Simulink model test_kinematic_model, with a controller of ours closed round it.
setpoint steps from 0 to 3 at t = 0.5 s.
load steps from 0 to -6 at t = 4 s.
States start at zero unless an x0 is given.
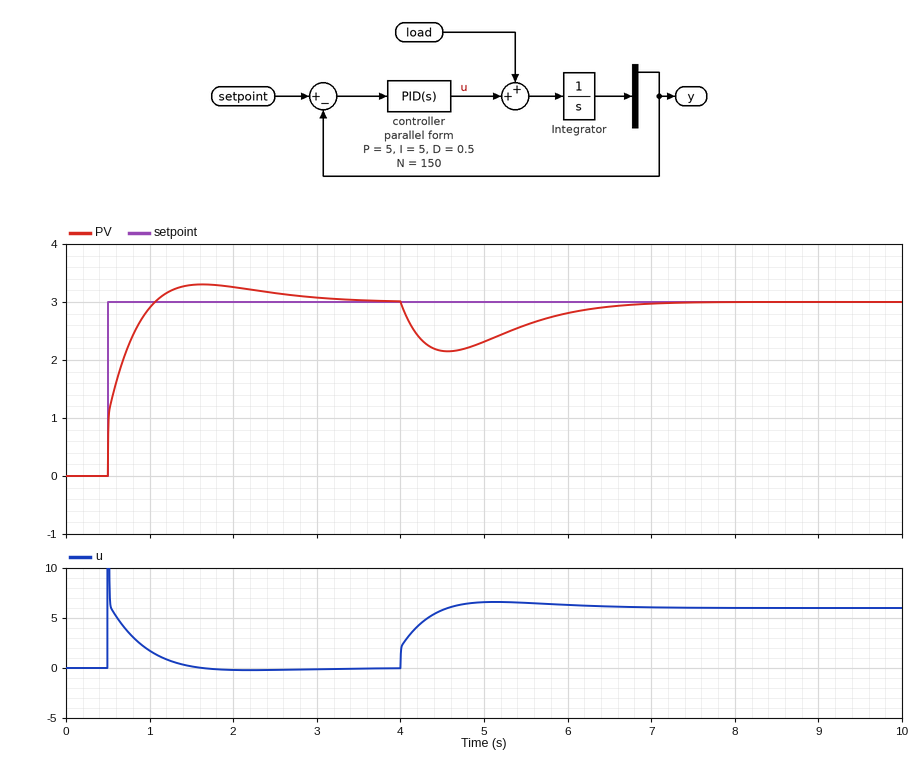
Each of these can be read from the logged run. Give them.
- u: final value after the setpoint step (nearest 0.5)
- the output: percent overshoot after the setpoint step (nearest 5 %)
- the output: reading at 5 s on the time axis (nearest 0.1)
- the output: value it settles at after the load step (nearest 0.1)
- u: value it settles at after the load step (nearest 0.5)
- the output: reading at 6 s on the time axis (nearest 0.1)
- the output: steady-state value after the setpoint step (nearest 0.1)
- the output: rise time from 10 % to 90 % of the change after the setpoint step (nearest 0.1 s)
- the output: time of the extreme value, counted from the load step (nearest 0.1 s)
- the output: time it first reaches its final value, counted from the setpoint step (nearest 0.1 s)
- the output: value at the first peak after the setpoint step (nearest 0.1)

0.0
10 %
2.3
3.0
6.0
2.8
3.0
0.4 s
0.6 s
0.6 s
3.3
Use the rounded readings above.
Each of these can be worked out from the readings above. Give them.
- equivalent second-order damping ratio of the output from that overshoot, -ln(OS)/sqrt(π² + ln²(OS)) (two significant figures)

0.59
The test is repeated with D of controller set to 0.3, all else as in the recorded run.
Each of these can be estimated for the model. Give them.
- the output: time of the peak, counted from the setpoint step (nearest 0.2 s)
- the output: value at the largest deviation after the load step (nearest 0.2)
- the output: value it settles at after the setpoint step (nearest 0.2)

1.0 s
2.2
3.0
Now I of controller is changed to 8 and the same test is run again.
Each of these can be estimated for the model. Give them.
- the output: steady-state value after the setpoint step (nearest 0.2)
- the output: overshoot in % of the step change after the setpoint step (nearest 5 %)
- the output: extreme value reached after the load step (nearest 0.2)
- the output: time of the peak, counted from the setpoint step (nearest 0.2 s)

3.0
15 %
2.2
1.0 s
